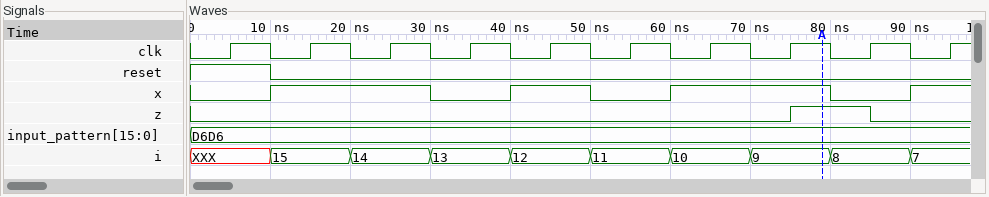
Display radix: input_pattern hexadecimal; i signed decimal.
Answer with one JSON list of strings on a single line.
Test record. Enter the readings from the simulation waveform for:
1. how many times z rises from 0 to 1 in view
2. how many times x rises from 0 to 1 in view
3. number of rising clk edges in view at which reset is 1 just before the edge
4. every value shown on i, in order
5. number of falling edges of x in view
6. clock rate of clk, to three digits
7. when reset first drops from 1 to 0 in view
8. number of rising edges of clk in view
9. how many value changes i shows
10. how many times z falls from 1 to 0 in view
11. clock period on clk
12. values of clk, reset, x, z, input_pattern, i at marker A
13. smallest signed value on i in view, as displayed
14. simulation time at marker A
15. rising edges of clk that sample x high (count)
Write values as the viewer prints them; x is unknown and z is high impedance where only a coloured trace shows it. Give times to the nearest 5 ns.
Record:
["1", "4", "1", "XXX, 15, 14, 13, 12, 11, 10, 9, 8, 7", "3", "100 MHz", "10 ns", "10", "9", "1", "10 ns", "clk=1, reset=0, x=1, z=1, input_pattern=D6D6, i=9", "7", "80 ns", "6"]
